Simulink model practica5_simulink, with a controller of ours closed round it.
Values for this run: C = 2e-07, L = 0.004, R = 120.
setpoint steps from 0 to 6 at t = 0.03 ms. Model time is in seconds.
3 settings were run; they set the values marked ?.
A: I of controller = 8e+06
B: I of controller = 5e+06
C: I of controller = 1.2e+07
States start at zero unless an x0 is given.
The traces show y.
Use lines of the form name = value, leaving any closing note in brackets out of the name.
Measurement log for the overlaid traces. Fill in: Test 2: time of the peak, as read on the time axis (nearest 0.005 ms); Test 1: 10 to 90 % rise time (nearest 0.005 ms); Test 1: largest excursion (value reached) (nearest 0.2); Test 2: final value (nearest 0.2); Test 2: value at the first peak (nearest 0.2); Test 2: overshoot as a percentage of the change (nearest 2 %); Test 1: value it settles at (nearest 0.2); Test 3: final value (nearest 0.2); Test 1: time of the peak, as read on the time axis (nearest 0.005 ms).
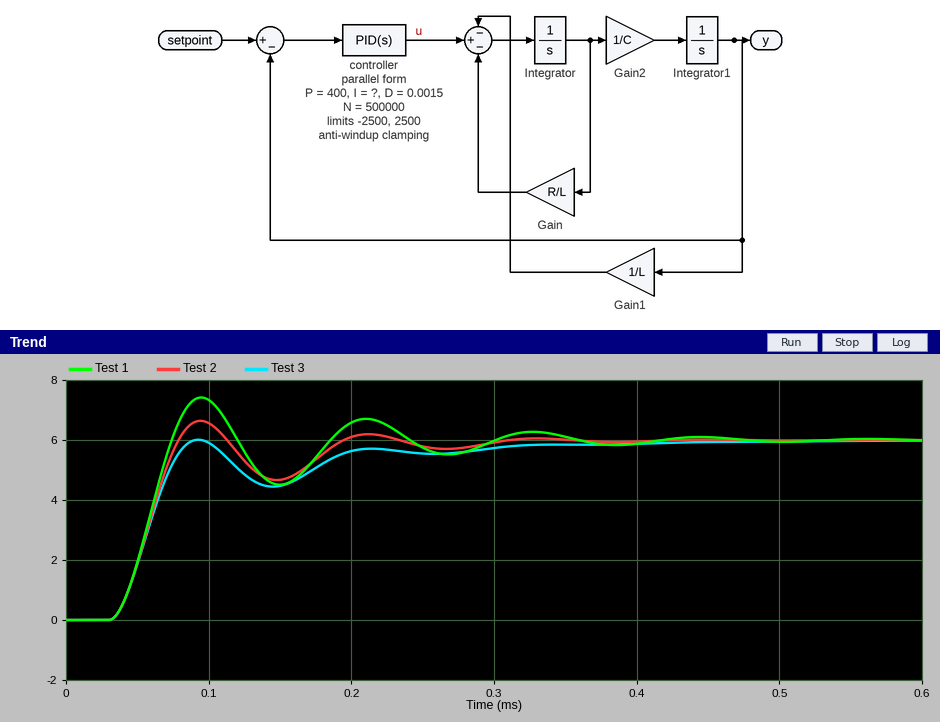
Test 2: time of the peak, as read on the time axis = 0.095 ms
Test 1: 10 to 90 % rise time = 0.030 ms
Test 1: largest excursion (value reached) = 7.4
Test 2: final value = 6.0
Test 2: value at the first peak = 6.6
Test 2: overshoot as a percentage of the change = 10 %
Test 1: value it settles at = 6.0
Test 3: final value = 6.0
Test 1: time of the peak, as read on the time axis = 0.095 ms
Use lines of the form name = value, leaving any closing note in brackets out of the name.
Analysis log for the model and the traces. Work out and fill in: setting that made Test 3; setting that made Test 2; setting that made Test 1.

setting that made Test 3 = B
setting that made Test 2 = A
setting that made Test 1 = C
